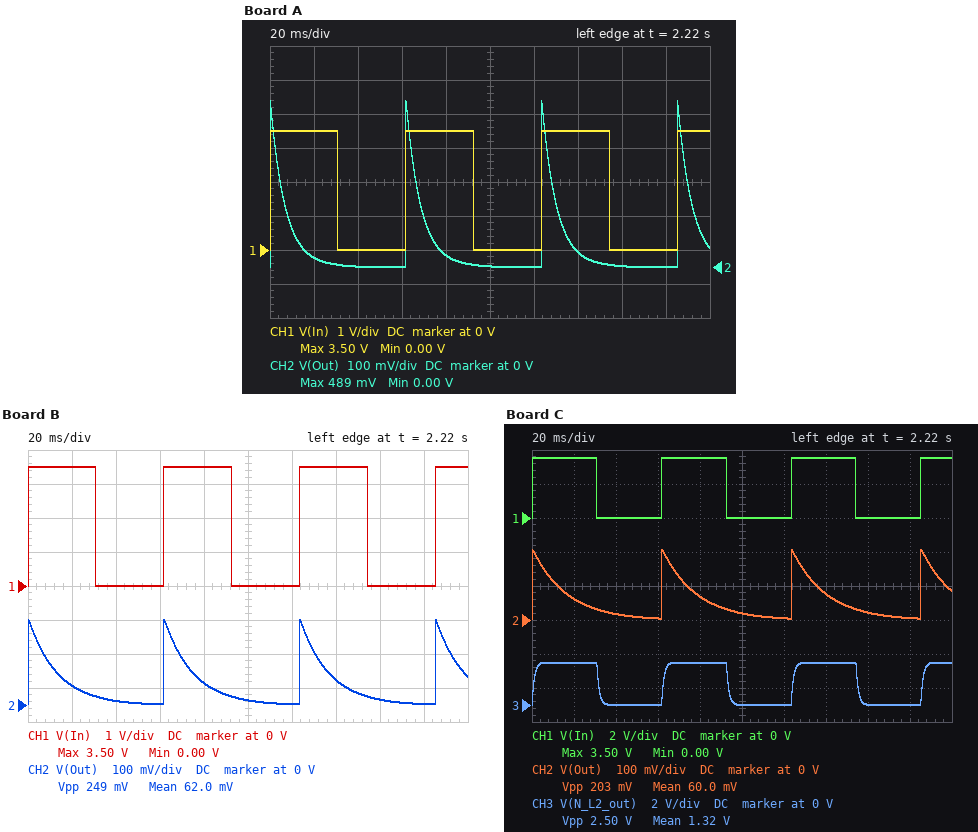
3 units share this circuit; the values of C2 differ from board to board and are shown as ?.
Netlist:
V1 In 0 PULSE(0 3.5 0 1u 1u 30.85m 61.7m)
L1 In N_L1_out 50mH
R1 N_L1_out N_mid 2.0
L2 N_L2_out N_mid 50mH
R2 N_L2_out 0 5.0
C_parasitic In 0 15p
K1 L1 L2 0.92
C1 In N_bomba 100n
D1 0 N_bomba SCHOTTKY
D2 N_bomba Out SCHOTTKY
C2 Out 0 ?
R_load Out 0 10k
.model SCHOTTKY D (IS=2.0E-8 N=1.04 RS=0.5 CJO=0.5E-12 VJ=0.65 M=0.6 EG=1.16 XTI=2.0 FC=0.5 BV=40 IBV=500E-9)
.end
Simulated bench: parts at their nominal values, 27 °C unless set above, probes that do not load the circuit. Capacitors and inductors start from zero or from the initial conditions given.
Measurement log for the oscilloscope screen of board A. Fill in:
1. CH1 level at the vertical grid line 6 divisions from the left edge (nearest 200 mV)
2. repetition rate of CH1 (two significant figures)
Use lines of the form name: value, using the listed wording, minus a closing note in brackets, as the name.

CH1 level at the vertical grid line 6 divisions from the left edge: 0 V
repetition rate of CH1: 16 Hz
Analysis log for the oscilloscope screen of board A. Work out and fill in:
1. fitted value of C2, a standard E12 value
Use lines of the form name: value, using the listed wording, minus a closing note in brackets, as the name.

fitted value of C2, a standard E12 value: 560 nF
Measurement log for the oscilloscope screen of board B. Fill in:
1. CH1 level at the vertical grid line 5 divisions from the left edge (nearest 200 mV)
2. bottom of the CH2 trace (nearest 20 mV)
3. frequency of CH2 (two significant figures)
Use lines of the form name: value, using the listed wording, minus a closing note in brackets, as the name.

CH1 level at the vertical grid line 5 divisions from the left edge: 0 V
bottom of the CH2 trace: 0 V
frequency of CH2: 16 Hz
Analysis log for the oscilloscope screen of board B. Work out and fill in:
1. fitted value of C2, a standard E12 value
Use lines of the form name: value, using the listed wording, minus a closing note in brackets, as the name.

fitted value of C2, a standard E12 value: 1.2 µF
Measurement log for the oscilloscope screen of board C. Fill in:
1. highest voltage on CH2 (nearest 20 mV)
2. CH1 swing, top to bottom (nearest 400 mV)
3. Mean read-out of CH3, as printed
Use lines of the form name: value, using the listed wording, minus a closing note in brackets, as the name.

highest voltage on CH2: 200 mV
CH1 swing, top to bottom: 3.6 V
Mean read-out of CH3, as printed: 1.32 V
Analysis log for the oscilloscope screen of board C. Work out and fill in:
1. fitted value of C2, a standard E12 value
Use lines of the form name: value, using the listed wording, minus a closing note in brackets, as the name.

fitted value of C2, a standard E12 value: 1.5 µF
